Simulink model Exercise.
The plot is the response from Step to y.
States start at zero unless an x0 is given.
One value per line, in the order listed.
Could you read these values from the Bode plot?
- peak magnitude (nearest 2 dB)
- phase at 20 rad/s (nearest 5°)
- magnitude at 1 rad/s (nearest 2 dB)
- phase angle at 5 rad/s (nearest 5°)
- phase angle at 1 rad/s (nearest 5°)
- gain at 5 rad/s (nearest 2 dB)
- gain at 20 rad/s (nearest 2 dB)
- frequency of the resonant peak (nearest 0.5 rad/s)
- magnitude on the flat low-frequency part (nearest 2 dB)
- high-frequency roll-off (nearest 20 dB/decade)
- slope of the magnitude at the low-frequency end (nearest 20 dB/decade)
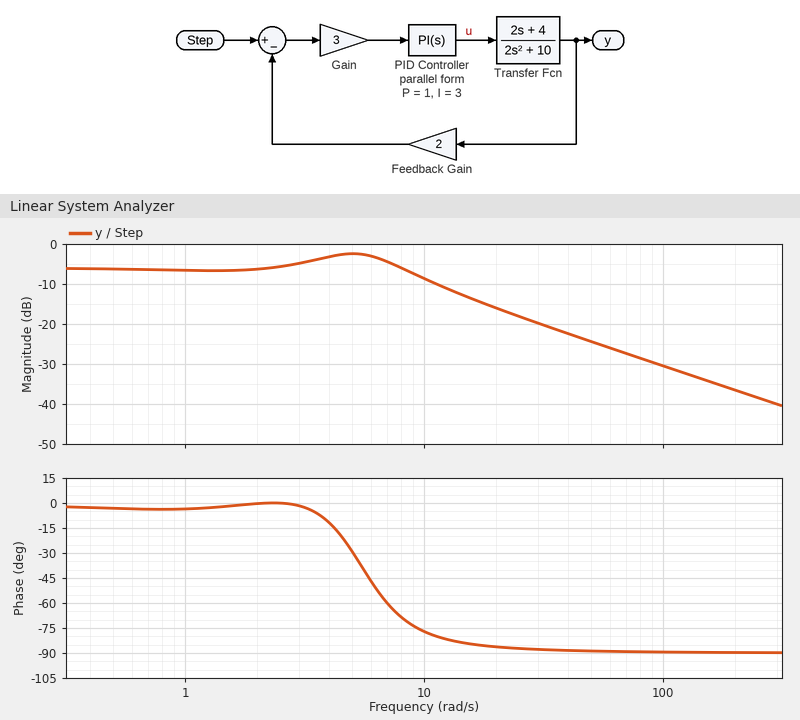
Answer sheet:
-2 dB
-85°
-6 dB
-30°
-5°
-2 dB
-16 dB
5.0 rad/s
-6 dB
-20 dB/decade
0 dB/decade
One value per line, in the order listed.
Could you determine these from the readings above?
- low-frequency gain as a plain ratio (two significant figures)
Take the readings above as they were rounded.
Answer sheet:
0.50
